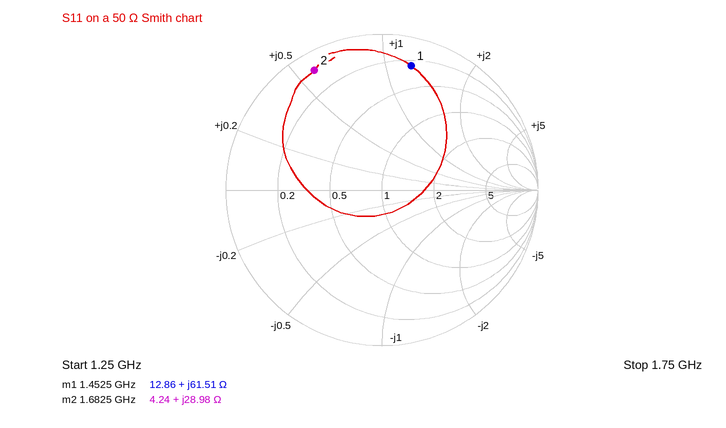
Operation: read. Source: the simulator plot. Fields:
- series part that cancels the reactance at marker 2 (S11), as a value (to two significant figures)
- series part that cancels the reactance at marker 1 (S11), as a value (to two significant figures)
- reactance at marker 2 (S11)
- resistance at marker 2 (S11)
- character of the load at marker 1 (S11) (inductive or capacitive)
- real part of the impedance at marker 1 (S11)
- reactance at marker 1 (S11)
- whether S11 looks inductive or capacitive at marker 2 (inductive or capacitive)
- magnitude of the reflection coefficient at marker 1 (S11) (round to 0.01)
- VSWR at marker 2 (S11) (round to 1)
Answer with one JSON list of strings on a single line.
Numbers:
["3.3 pF", "1.8 pF", "+28.98 Ω", "4.24 Ω", "inductive", "12.86 Ω", "+61.51 Ω", "inductive", "0.82", "16"]
